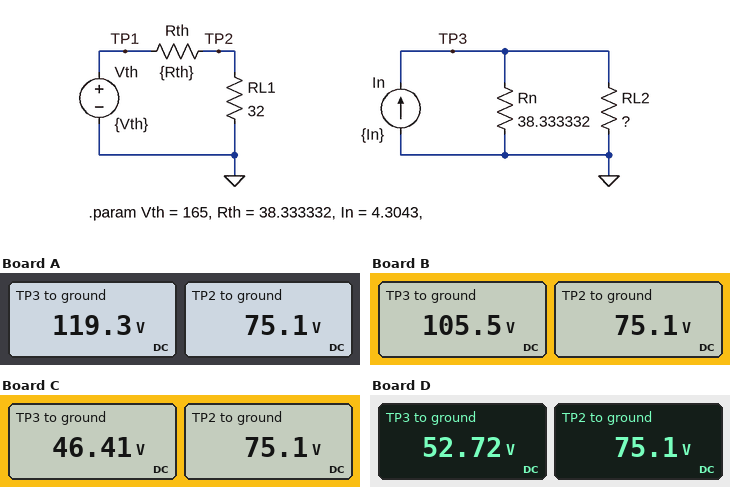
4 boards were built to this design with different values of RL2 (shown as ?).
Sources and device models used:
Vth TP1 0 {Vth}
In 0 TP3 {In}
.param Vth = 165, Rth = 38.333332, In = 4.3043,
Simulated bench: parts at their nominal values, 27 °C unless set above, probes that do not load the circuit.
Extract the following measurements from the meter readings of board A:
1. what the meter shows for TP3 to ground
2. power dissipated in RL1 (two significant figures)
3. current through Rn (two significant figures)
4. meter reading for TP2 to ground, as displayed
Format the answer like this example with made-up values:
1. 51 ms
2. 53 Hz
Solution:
1. 119.3 V
2. 180 W
3. 3.1 A
4. 75.1 V
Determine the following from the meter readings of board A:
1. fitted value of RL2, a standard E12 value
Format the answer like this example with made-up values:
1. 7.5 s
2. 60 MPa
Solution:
1. 100 Ω
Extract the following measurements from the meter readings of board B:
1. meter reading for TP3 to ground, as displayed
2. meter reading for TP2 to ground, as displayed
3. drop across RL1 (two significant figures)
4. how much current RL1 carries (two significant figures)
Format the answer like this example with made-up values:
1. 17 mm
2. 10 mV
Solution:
1. 105.5 V
2. 75.1 V
3. 75 V
4. 2.3 A
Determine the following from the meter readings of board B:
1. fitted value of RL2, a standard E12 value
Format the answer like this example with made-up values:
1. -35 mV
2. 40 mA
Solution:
1. 68 Ω
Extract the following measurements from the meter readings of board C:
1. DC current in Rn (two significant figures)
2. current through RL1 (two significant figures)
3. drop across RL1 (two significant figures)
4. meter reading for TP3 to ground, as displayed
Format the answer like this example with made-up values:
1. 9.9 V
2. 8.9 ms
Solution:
1. 1.2 A
2. 2.3 A
3. 75 V
4. 46.41 V
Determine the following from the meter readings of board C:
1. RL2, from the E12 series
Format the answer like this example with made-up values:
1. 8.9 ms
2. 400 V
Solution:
1. 15 Ω
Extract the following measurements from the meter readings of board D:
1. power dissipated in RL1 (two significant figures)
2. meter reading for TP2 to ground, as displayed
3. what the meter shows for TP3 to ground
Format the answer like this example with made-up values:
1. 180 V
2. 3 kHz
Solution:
1. 180 W
2. 75.1 V
3. 52.72 V
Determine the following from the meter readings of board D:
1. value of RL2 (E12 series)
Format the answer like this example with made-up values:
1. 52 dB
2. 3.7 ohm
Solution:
1. 18 Ω
